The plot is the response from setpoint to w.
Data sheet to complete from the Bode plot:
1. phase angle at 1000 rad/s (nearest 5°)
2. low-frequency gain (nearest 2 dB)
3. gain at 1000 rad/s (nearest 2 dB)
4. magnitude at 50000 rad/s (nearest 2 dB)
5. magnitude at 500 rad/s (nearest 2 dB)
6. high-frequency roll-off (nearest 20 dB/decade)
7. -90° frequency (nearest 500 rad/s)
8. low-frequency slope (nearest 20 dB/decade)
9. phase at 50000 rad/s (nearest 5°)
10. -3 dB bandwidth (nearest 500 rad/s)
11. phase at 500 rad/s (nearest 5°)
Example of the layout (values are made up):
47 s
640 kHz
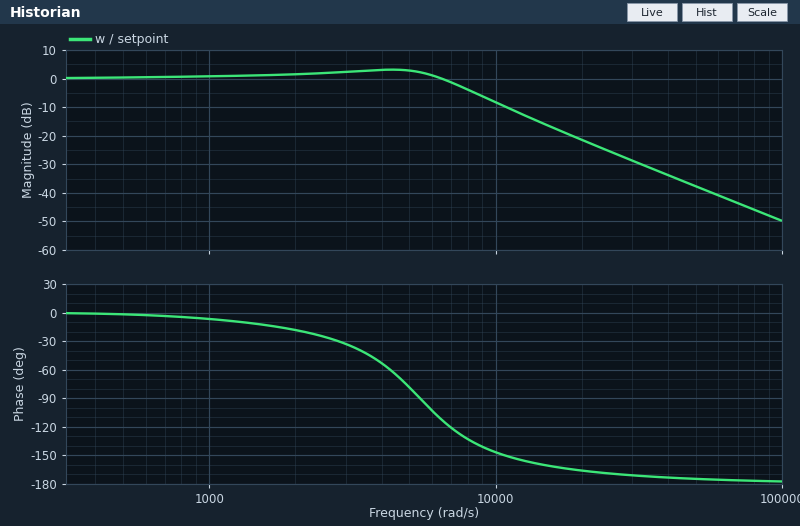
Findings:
-5°
0 dB
0 dB
-38 dB
0 dB
-40 dB/decade
5500 rad/s
0 dB/decade
-175°
7500 rad/s
0°
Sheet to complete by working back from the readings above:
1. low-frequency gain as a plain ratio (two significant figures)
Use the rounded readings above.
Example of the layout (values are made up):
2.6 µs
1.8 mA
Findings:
1.0
